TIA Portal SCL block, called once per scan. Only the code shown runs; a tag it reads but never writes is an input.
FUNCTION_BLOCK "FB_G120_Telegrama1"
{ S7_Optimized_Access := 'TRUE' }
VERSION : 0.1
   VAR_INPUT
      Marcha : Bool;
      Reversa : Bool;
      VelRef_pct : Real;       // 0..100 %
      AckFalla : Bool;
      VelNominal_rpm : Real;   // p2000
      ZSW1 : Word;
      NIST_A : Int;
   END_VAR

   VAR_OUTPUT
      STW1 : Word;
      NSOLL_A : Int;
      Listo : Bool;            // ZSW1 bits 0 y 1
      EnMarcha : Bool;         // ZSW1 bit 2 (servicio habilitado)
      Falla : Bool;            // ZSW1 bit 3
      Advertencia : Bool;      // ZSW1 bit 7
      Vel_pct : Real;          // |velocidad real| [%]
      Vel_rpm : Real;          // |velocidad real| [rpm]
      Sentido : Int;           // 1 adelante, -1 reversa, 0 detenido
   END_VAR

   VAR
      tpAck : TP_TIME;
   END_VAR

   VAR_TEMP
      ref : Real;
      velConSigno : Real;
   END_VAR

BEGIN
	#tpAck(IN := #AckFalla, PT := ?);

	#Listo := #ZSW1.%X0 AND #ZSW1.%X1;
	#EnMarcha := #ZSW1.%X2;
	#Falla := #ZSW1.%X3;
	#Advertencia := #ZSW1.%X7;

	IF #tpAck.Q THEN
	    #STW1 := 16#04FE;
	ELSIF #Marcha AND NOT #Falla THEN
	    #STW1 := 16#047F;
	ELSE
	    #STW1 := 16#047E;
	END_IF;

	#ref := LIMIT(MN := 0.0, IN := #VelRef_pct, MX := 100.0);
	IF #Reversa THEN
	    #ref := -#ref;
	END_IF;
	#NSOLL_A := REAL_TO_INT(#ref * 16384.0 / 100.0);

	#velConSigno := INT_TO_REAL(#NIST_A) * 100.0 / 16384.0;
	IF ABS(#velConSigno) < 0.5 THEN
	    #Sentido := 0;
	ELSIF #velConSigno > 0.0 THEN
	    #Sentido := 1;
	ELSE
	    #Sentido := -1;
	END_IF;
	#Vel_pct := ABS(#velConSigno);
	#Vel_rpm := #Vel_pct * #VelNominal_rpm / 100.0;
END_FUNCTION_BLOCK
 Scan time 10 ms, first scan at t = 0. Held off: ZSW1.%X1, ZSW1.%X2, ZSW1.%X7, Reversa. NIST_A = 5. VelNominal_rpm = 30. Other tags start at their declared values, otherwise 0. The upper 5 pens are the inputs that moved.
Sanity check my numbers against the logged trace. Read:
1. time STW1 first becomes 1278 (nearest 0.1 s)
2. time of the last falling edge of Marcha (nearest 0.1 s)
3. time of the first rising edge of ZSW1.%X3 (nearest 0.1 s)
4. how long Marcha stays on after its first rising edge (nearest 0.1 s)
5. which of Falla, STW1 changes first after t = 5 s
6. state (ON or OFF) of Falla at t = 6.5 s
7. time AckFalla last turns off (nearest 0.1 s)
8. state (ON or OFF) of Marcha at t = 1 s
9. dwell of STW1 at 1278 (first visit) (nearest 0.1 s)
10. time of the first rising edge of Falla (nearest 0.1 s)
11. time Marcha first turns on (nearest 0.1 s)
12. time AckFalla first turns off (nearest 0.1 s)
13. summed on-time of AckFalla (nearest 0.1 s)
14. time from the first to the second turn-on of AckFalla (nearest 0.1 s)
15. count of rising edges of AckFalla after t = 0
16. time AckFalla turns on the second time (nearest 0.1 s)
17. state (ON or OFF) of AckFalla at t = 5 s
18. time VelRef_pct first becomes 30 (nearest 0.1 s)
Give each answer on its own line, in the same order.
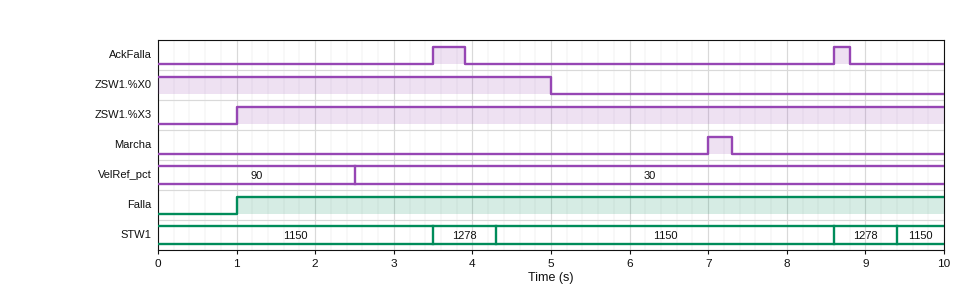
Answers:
3.5 s
7.3 s
1.0 s
0.3 s
STW1
ON
8.8 s
OFF
0.8 s
1.0 s
7.0 s
3.9 s
0.6 s
5.1 s
2
8.6 s
OFF
2.5 s
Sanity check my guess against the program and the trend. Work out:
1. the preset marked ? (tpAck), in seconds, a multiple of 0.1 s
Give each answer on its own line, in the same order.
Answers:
0.8 s
